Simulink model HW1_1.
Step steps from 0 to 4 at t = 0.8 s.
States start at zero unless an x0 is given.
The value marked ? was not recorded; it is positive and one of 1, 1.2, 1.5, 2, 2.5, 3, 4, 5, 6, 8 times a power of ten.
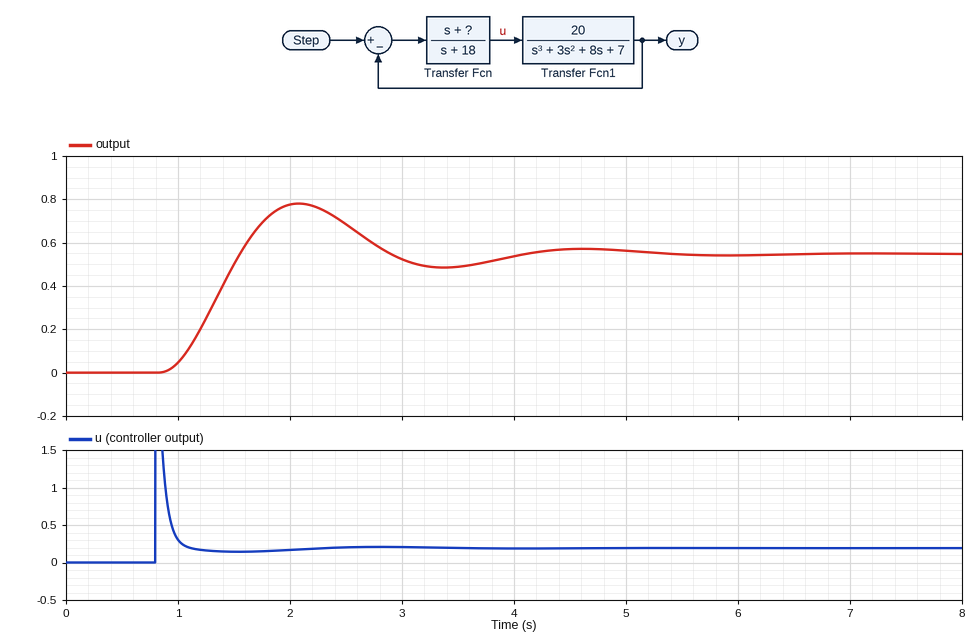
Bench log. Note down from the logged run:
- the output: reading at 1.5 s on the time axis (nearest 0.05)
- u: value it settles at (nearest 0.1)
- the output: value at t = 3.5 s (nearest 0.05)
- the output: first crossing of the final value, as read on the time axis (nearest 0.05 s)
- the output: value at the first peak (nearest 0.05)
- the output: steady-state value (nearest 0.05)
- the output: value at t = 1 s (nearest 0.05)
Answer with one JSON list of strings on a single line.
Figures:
["0.50", "0.2", "0.50", "1.55 s", "0.80", "0.55", "0.05"]
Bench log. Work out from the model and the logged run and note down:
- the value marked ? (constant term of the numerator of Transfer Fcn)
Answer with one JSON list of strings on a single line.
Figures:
["1"]
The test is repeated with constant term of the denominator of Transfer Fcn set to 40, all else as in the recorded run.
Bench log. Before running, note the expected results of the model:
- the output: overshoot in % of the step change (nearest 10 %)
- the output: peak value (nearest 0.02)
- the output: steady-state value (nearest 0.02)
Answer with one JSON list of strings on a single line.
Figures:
["40 %", "0.38", "0.26"]
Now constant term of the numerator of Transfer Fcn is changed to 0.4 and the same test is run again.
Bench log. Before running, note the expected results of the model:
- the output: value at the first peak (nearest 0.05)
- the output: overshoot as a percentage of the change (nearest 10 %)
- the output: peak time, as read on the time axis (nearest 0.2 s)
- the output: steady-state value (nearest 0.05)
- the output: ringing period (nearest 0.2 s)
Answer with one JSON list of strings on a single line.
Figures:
["0.60", "150 %", "2.0 s", "0.25", "2.6 s"]
